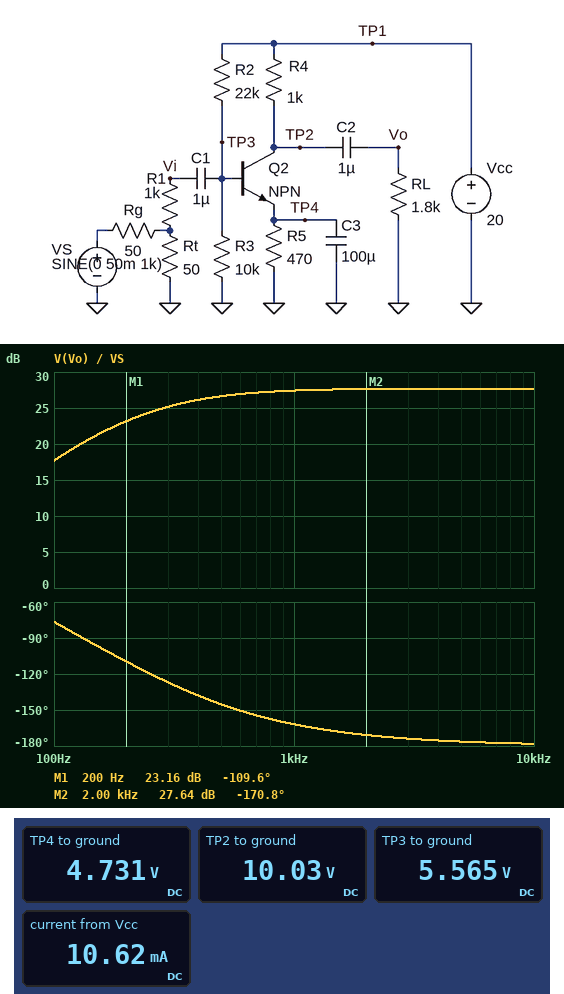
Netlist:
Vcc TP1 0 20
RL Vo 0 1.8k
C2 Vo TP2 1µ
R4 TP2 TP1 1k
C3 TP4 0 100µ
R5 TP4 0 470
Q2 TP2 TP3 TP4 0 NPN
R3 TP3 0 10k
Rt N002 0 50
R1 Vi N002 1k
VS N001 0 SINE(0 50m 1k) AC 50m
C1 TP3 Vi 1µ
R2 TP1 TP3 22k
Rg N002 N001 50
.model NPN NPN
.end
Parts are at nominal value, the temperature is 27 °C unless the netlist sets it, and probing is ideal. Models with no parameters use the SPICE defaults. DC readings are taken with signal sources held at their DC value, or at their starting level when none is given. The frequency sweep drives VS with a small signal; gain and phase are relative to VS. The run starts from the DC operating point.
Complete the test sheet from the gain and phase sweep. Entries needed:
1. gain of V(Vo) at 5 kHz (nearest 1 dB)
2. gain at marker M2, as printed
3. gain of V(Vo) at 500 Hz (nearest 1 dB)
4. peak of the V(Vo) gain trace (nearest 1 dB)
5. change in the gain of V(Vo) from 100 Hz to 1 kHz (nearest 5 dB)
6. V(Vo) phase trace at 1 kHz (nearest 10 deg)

28 dB
27.64 dB
27 dB
28 dB
10 dB
-160 deg
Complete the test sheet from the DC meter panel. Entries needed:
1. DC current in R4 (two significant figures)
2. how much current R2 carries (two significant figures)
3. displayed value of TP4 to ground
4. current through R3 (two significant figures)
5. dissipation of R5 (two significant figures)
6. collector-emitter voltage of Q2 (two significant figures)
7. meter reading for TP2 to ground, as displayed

10 mA
660 µA
4.731 V
560 µA
48 mW
5.3 V
10.03 V
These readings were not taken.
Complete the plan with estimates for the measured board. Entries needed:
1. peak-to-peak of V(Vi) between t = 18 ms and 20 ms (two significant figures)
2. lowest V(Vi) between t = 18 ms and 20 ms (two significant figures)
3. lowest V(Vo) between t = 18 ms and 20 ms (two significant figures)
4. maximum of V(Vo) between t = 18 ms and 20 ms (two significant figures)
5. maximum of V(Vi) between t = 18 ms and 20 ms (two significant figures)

15 mV
-7.5 mV
-1.2 V
1.2 V
7.7 mV
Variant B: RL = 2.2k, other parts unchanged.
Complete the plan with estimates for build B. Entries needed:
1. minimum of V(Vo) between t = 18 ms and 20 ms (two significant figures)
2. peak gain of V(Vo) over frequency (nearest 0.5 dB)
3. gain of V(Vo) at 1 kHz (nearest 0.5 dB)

-1.3 V
28.5 dB
28.0 dB
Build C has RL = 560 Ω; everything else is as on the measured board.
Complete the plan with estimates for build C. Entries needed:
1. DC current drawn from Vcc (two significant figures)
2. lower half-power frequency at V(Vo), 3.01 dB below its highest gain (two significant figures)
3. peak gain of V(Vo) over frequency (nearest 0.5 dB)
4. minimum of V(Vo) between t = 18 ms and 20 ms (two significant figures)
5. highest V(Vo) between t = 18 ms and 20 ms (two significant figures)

11 mA
290 Hz
22.5 dB
-660 mV
650 mV
